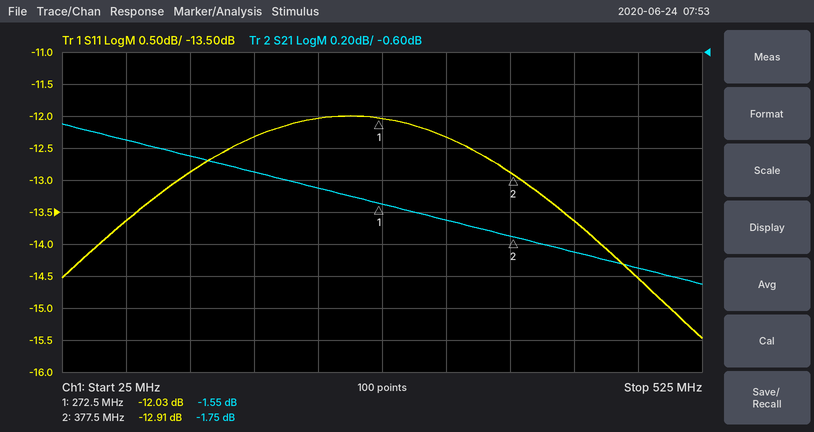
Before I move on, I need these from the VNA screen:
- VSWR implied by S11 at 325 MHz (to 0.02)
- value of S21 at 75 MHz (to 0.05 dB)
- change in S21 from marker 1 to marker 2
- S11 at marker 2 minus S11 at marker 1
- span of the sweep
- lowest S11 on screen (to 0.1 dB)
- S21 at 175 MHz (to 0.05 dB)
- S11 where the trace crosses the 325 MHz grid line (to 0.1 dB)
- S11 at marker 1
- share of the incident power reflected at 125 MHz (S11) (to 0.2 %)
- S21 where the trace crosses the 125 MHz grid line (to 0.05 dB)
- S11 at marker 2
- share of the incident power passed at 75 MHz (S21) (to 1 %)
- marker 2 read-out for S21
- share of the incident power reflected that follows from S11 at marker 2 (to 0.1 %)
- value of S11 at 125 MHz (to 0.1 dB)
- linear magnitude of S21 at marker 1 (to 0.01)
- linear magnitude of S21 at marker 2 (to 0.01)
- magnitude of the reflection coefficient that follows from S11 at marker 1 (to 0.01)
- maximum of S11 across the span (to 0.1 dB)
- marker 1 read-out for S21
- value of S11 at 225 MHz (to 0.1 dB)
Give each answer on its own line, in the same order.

1.64
-1.15 dB
-0.20 dB
-0.88 dB
500 MHz
-15.5 dB
-1.35 dB
-12.3 dB
-12.03 dB
5.2 %
-1.25 dB
-12.91 dB
77 %
-1.75 dB
5.1 %
-12.9 dB
0.84
0.82
0.25
-12.0 dB
-1.55 dB
-12.0 dB
